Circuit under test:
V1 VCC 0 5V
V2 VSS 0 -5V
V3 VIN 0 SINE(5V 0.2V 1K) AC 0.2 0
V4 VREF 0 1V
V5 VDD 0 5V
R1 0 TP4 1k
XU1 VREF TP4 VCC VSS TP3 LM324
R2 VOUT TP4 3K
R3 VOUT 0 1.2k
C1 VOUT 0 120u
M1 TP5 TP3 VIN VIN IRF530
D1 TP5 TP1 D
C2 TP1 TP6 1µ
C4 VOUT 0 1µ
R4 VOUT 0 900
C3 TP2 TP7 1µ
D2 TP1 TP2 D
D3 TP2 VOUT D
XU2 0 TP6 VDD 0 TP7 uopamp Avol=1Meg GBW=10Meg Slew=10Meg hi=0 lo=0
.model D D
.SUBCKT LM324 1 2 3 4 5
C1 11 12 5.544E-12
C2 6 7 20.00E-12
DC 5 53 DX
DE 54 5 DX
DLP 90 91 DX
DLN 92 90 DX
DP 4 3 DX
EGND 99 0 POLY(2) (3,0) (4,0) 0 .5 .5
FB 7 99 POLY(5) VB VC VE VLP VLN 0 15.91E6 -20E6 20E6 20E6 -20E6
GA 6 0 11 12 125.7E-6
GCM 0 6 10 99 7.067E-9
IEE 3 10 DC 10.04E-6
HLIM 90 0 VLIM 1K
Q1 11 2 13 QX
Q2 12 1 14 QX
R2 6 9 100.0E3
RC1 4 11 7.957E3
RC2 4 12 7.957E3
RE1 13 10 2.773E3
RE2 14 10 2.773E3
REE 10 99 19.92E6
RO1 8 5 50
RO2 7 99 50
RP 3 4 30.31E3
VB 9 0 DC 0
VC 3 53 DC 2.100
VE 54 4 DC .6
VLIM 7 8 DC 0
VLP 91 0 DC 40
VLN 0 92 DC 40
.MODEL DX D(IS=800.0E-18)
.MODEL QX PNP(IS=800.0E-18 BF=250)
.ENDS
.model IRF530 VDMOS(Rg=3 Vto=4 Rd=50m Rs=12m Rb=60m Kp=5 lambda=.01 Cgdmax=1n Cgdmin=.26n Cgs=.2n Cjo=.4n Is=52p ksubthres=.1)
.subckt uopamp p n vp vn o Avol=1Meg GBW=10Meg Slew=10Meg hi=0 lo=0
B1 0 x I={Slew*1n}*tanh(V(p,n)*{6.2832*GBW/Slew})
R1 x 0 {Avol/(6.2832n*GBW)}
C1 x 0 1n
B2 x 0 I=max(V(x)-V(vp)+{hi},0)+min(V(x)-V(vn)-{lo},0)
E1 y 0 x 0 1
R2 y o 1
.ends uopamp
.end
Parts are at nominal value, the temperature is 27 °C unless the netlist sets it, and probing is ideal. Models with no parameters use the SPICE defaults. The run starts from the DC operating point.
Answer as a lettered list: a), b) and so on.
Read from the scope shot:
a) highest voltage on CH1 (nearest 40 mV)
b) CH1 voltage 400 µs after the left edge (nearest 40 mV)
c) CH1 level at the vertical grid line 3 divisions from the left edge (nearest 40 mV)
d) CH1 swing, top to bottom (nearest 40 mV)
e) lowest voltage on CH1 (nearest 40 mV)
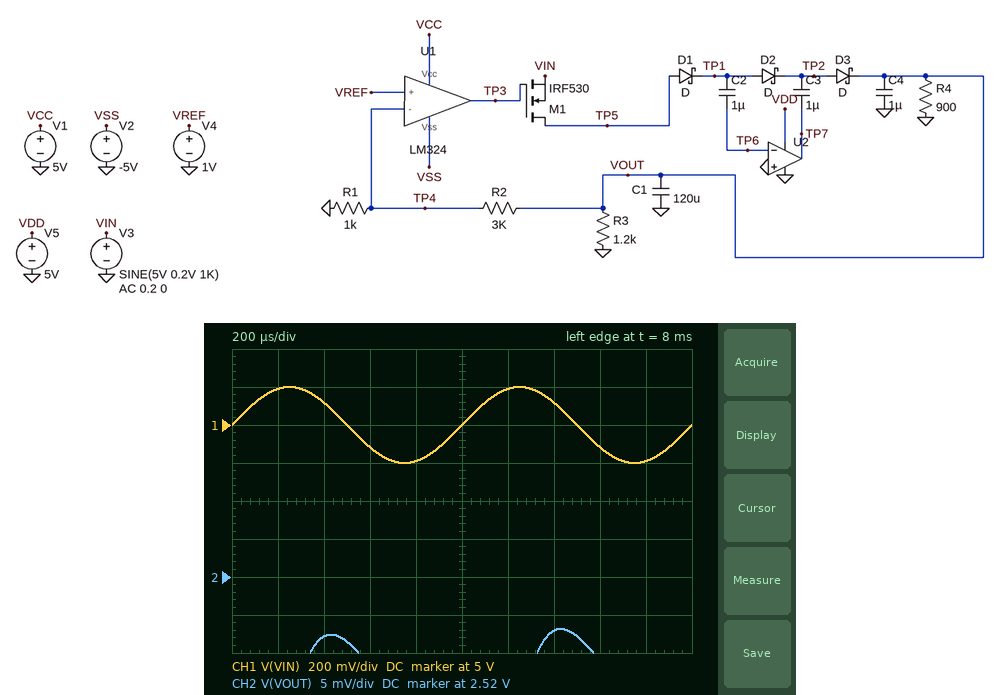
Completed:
a) 5.20 V
b) 5.12 V
c) 4.88 V
d) 400 mV
e) 4.80 V
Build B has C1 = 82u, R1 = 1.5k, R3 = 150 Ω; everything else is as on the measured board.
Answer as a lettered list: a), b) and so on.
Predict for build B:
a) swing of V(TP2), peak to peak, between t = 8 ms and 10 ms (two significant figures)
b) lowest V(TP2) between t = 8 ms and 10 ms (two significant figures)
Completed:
a) 140 mV
b) 3.0 V
